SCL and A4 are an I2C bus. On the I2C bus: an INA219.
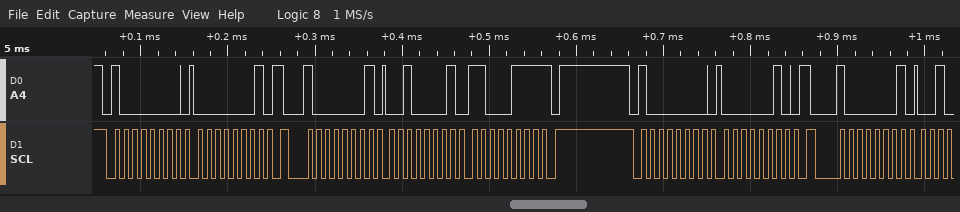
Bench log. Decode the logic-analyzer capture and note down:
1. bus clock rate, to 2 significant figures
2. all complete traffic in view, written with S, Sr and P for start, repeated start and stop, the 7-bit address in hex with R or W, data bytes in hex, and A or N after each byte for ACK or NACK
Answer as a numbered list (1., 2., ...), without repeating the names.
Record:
1. 100 kHz
2. S 40W A 01 A Sr 40R A 21 A C7 N P S 40W A 02 A Sr 40R A
